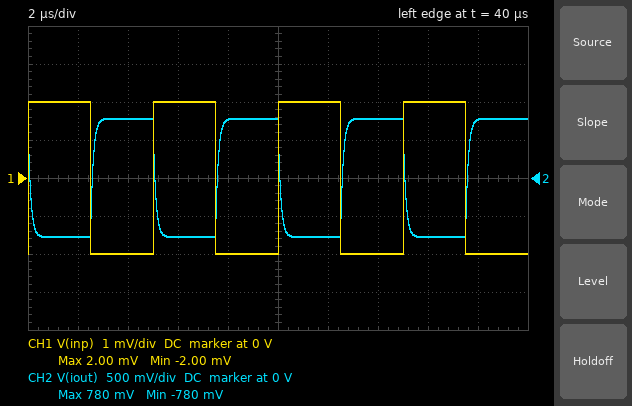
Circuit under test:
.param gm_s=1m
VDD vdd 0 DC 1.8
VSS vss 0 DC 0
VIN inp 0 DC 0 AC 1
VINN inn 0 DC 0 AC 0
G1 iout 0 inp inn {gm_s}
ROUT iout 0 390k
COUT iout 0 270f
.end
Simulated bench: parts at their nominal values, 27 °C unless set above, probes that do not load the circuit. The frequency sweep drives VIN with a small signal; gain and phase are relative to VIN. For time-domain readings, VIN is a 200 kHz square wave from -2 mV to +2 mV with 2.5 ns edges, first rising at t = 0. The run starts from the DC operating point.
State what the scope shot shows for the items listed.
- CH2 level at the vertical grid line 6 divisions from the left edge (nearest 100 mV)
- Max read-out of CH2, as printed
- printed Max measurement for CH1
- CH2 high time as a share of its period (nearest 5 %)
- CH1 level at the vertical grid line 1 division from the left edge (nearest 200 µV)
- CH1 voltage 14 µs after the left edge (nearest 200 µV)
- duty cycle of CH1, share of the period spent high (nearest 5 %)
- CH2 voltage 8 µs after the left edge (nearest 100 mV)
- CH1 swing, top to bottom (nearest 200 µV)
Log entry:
-800 mV
780 mV
2.00 mV
50 %
2.0 mV
-2.0 mV
50 %
800 mV
4.0 mV
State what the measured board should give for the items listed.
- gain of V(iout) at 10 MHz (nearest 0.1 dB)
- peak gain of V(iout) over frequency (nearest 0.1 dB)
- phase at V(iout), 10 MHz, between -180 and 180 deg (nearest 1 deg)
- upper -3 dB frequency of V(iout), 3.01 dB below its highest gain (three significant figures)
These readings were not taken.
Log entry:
35.3 dB
51.8 dB
99 deg
1.51 MHz
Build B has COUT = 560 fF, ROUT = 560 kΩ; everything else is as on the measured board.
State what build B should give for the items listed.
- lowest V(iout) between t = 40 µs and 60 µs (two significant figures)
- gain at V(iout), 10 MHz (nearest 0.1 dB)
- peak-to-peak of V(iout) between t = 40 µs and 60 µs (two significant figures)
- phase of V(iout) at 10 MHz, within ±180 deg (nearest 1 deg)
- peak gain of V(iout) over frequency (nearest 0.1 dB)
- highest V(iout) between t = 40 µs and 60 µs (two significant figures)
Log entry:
-1.1 V
29.1 dB
2.2 V
93 deg
55.0 dB
1.1 V
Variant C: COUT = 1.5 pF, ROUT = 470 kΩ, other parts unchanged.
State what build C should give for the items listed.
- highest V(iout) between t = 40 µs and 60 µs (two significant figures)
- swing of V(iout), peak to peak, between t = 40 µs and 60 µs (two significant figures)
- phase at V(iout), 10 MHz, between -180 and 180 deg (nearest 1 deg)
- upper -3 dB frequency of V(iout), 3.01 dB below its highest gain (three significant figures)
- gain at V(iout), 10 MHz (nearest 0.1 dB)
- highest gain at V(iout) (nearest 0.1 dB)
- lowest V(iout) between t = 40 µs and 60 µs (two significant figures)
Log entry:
890 mV
1.8 V
91 deg
226 kHz
20.5 dB
53.4 dB
-890 mV
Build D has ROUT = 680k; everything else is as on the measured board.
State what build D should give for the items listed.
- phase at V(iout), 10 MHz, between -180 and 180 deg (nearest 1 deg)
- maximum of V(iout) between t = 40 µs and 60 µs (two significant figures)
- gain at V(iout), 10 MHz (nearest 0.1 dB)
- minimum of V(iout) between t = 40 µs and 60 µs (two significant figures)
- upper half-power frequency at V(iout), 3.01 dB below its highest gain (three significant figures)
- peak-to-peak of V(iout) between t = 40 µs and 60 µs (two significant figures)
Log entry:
95 deg
1.4 V
35.4 dB
-1.4 V
867 kHz
2.7 V
